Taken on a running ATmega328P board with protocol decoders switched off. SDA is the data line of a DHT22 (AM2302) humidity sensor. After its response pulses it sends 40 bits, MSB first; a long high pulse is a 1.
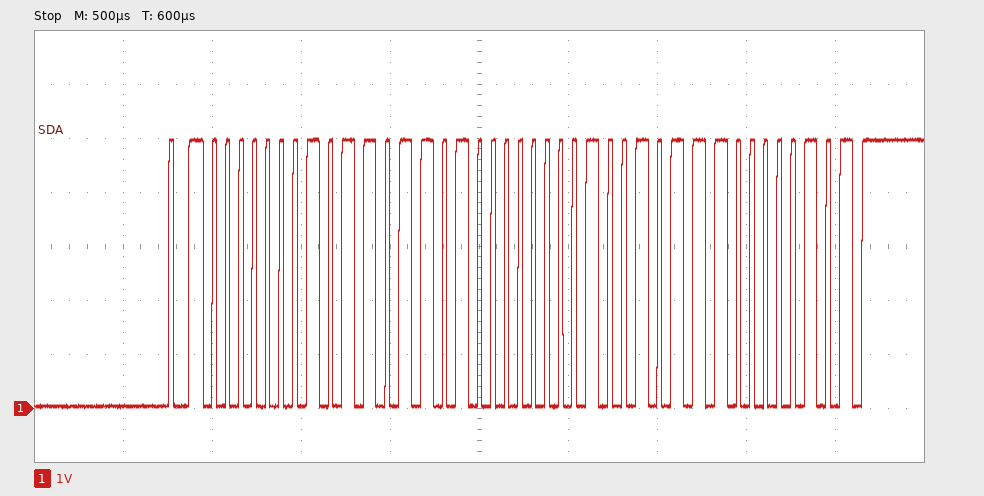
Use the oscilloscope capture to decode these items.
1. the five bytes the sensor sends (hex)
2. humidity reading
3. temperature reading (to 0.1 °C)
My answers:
01 6D 00 97 05
36.5 %
15.1 °C
